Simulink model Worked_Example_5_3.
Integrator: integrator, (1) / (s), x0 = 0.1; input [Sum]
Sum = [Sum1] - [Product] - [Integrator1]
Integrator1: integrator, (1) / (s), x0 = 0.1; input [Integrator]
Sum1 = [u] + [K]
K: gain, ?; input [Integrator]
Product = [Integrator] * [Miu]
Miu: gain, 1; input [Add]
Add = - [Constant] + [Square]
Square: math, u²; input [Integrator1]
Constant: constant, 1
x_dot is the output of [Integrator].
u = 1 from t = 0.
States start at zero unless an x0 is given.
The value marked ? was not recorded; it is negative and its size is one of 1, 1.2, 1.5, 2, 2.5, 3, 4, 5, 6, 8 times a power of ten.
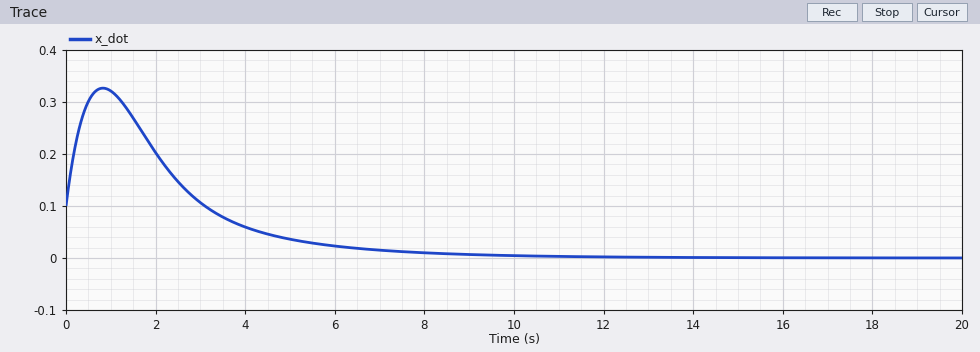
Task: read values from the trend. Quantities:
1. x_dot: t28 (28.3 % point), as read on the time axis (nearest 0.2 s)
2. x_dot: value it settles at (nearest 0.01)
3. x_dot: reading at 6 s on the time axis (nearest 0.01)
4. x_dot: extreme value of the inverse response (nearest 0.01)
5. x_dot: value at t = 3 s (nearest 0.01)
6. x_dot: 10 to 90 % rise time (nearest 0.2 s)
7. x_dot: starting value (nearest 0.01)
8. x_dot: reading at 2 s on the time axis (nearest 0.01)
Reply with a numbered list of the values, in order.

1. 3.6 s
2. 0.00
3. 0.02
4. 0.33
5. 0.11
6. 4.8 s
7. 0.10
8. 0.20
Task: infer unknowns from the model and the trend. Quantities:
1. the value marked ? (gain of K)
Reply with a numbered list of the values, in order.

1. -3
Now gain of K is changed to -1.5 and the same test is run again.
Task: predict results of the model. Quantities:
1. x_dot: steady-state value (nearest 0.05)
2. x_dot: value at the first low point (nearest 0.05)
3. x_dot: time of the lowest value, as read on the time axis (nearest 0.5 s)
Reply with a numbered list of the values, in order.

1. 0.00
2. -0.05
3. 4.0 s
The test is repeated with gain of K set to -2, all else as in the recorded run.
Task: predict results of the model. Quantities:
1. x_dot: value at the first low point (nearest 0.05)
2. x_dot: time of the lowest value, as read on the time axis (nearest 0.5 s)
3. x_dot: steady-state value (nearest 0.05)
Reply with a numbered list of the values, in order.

1. 0.00
2. 5.5 s
3. 0.00
